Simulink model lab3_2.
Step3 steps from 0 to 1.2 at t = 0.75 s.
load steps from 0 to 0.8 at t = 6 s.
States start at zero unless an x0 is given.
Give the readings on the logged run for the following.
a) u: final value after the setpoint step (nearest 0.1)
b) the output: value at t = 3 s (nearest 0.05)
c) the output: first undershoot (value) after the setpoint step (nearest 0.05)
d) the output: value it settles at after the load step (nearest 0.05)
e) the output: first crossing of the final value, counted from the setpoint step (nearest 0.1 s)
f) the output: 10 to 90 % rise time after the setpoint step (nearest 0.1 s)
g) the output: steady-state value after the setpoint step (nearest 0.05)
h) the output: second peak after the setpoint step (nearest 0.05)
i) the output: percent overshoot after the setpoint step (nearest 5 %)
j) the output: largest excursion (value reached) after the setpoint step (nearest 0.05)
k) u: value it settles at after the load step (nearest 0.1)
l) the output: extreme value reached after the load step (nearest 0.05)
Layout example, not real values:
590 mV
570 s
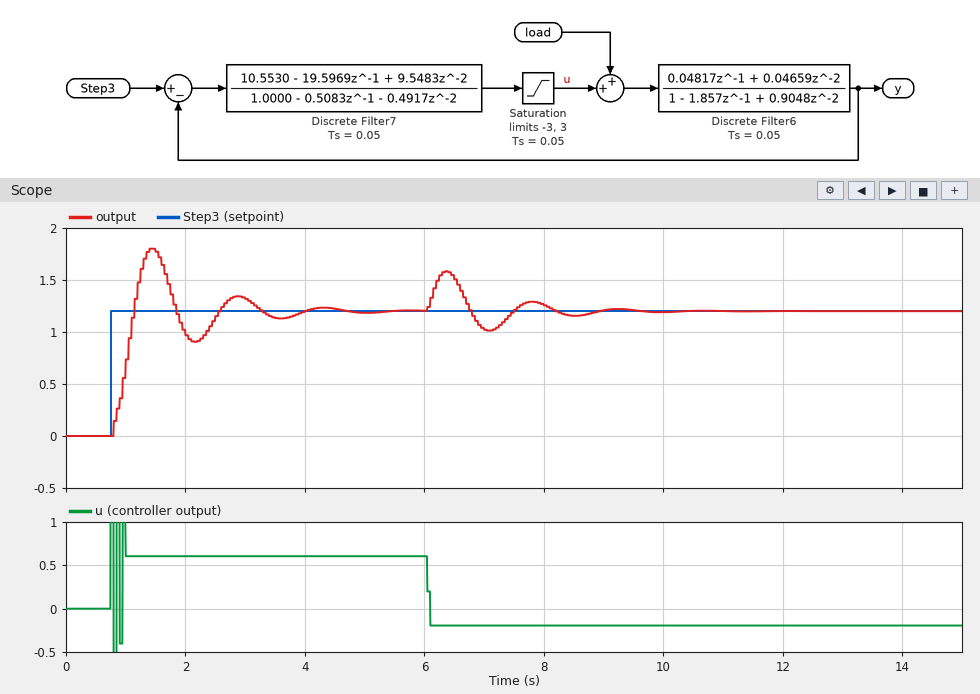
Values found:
0.6
1.30
0.90
1.20
0.4 s
0.3 s
1.20
1.35
50 %
1.80
-0.2
1.60
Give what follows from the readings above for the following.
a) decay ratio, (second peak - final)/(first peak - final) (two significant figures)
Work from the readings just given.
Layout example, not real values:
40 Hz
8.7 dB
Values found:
0.25
